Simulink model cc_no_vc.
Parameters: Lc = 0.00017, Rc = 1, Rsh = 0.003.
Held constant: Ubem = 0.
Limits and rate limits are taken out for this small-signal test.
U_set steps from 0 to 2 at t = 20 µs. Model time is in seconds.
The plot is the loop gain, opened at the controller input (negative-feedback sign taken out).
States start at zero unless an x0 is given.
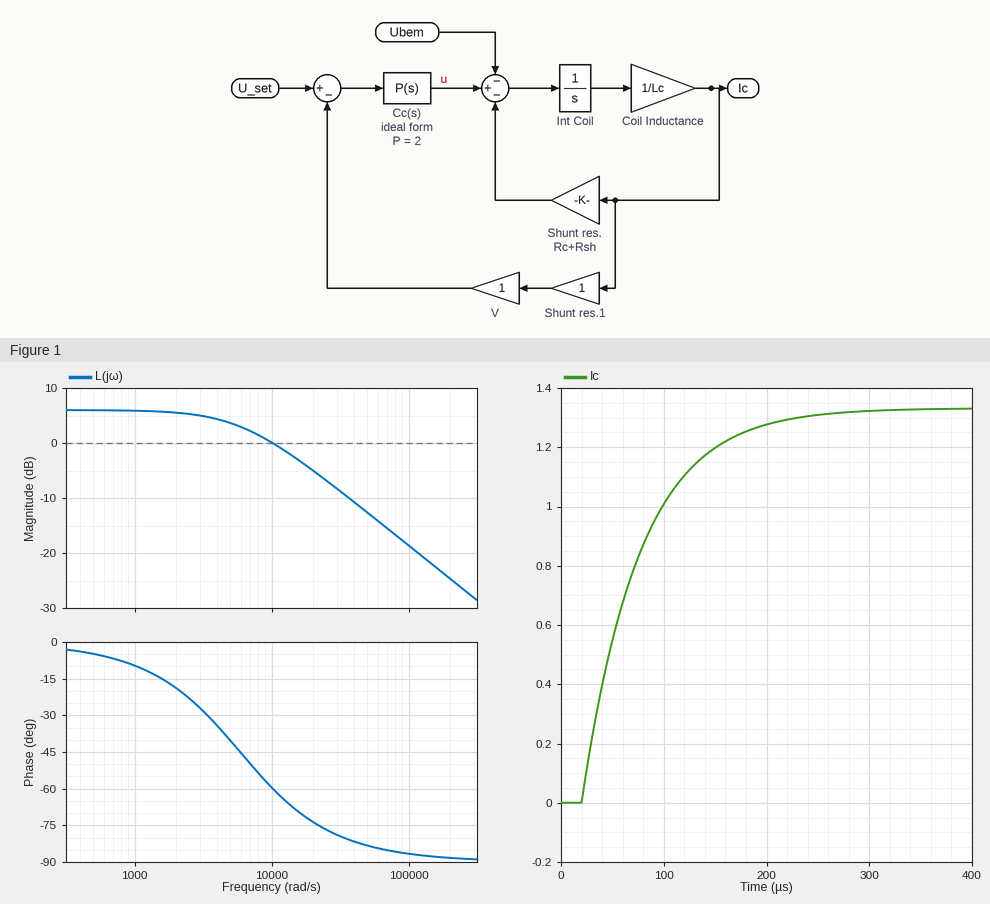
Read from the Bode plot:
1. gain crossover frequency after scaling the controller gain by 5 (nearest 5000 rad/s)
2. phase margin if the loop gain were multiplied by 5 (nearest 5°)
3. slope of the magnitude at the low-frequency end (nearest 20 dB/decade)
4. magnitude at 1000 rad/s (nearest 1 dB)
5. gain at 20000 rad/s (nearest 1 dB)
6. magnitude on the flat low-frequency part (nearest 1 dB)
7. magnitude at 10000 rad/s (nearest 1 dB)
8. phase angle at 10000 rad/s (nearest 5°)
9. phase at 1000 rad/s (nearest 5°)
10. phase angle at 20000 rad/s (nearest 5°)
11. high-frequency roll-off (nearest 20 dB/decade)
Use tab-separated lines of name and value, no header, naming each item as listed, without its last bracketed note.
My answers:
gain crossover frequency after scaling the controller gain by 5	60000 rad/s
phase margin if the loop gain were multiplied by 5	95°
slope of the magnitude at the low-frequency end	0 dB/decade
magnitude at 1000 rad/s	6 dB
gain at 20000 rad/s	-5 dB
magnitude on the flat low-frequency part	6 dB
magnitude at 10000 rad/s	0 dB
phase angle at 10000 rad/s	-60°
phase at 1000 rad/s	-10°
phase angle at 20000 rad/s	-75°
high-frequency roll-off	-20 dB/decade
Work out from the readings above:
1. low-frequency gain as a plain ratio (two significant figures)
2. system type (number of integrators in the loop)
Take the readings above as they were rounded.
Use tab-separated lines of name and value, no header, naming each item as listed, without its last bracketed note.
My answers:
low-frequency gain as a plain ratio	2.0
system type	0
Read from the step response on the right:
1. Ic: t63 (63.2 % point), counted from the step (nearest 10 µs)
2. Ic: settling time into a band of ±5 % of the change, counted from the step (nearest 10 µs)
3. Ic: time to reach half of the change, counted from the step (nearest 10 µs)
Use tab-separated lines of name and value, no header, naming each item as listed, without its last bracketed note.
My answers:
Ic: t63 (63.2 % point), counted from the step	60 µs
Ic: settling time into a band of ±5 % of the change, counted from the step	170 µs
Ic: time to reach half of the change, counted from the step	40 µs
